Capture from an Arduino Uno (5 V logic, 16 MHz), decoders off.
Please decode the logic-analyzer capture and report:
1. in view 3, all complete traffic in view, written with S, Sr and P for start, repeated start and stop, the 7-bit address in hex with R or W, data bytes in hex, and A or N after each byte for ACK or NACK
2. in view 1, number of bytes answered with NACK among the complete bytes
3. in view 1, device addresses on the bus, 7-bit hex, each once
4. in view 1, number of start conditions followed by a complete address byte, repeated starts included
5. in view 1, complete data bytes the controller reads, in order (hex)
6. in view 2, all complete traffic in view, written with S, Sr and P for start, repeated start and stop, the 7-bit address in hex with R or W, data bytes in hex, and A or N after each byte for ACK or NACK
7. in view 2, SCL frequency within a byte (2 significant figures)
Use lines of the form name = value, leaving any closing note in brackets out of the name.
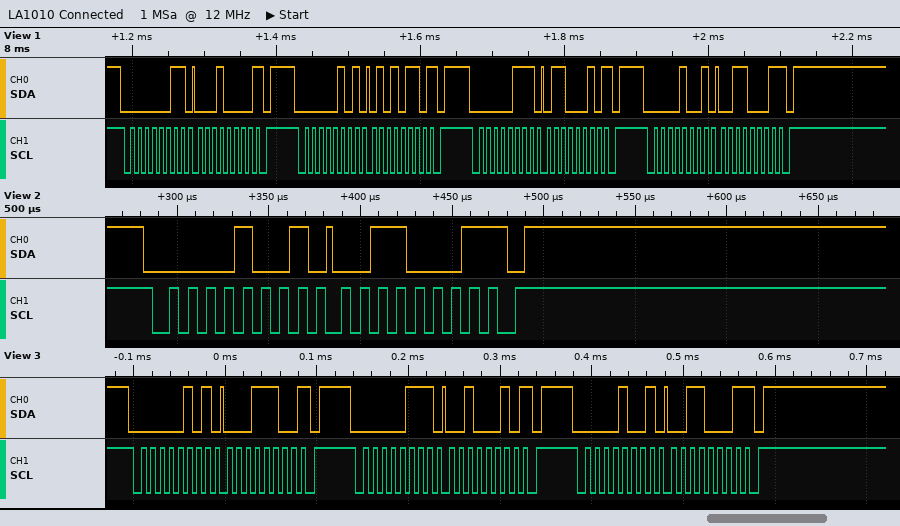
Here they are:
in view 3, all complete traffic in view, written with S, Sr and P for start, repeated start and stop, the 7-bit address in hex with R or W, data bytes in hex, and A or N after each byte for ACK or NACK = S 02R A 1C N P S 03R A 22 N P S 04R A 31 N P
in view 1, number of bytes answered with NACK among the complete bytes = 4
in view 1, device addresses on the bus, 7-bit hex, each once = 0x01 0x02 0x03 0x04
in view 1, number of start conditions followed by a complete address byte, repeated starts included = 4
in view 1, complete data bytes the controller reads, in order = 10 56 62 31
in view 2, all complete traffic in view, written with S, Sr and P for start, repeated start and stop, the 7-bit address in hex with R or W, data bytes in hex, and A or N after each byte for ACK or NACK = S 04R A 31 N P
in view 2, SCL frequency within a byte = 100 kHz
